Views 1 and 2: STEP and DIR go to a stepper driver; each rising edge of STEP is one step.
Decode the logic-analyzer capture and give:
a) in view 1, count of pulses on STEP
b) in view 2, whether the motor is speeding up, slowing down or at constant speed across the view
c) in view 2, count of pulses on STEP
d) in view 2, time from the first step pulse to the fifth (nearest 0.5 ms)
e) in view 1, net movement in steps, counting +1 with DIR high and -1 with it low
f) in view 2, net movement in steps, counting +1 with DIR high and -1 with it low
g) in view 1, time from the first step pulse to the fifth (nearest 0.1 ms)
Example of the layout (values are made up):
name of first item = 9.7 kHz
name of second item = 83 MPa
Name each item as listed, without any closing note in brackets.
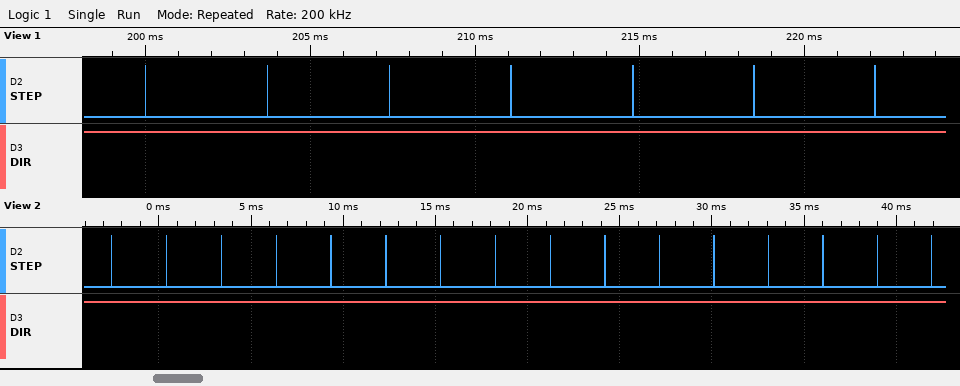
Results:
in view 1, count of pulses on STEP = 7
in view 2, whether the motor is speeding up, slowing down or at constant speed across the view = constant speed
in view 2, count of pulses on STEP = 16
in view 2, time from the first step pulse to the fifth = 12.0 ms
in view 1, net movement in steps, counting +1 with DIR high and -1 with it low = +7
in view 2, net movement in steps, counting +1 with DIR high and -1 with it low = +16
in view 1, time from the first step pulse to the fifth = 14.8 ms
